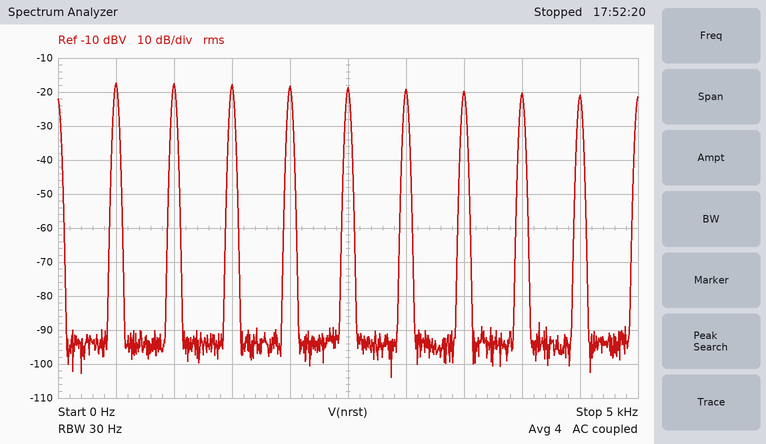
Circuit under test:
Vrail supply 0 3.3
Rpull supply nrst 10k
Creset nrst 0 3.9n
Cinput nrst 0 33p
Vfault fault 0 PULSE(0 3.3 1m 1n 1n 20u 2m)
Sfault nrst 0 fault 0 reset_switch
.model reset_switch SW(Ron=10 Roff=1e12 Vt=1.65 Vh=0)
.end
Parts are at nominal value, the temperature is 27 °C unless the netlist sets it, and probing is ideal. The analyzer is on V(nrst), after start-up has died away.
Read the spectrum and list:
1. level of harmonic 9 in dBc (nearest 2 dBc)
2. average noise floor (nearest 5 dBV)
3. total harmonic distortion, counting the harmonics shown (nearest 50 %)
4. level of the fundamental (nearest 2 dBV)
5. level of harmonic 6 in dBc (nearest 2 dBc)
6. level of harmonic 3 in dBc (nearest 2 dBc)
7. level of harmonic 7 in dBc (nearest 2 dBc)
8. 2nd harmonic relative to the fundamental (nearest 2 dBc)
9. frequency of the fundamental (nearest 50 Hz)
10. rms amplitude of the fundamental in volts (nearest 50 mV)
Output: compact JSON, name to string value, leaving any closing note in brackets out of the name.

{"level of harmonic 9 in dBc": "-4 dBc", "average noise floor": "-95 dBV", "total harmonic distortion, counting the harmonics shown": "250 %", "level of the fundamental": "-18 dBV", "level of harmonic 6 in dBc": "-2 dBc", "level of harmonic 3 in dBc": "0 dBc", "level of harmonic 7 in dBc": "-2 dBc", "2nd harmonic relative to the fundamental": "0 dBc", "frequency of the fundamental": "500 Hz", "rms amplitude of the fundamental in volts": "150 mV"}
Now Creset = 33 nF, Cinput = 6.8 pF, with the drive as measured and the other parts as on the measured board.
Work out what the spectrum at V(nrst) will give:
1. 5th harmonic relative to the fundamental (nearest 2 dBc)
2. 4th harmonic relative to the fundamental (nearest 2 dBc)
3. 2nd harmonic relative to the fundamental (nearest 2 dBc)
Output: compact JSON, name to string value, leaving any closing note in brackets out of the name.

{"5th harmonic relative to the fundamental": "-12 dBc", "4th harmonic relative to the fundamental": "-10 dBc", "2nd harmonic relative to the fundamental": "-4 dBc"}
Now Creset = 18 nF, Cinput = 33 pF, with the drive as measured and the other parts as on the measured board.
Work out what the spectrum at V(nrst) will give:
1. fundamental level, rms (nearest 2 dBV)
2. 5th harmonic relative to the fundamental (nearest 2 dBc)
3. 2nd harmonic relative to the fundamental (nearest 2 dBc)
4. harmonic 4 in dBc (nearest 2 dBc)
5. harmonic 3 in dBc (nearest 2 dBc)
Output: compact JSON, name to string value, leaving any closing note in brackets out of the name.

{"fundamental level, rms": "-8 dBV", "5th harmonic relative to the fundamental": "-8 dBc", "2nd harmonic relative to the fundamental": "-2 dBc", "harmonic 4 in dBc": "-6 dBc", "harmonic 3 in dBc": "-4 dBc"}
